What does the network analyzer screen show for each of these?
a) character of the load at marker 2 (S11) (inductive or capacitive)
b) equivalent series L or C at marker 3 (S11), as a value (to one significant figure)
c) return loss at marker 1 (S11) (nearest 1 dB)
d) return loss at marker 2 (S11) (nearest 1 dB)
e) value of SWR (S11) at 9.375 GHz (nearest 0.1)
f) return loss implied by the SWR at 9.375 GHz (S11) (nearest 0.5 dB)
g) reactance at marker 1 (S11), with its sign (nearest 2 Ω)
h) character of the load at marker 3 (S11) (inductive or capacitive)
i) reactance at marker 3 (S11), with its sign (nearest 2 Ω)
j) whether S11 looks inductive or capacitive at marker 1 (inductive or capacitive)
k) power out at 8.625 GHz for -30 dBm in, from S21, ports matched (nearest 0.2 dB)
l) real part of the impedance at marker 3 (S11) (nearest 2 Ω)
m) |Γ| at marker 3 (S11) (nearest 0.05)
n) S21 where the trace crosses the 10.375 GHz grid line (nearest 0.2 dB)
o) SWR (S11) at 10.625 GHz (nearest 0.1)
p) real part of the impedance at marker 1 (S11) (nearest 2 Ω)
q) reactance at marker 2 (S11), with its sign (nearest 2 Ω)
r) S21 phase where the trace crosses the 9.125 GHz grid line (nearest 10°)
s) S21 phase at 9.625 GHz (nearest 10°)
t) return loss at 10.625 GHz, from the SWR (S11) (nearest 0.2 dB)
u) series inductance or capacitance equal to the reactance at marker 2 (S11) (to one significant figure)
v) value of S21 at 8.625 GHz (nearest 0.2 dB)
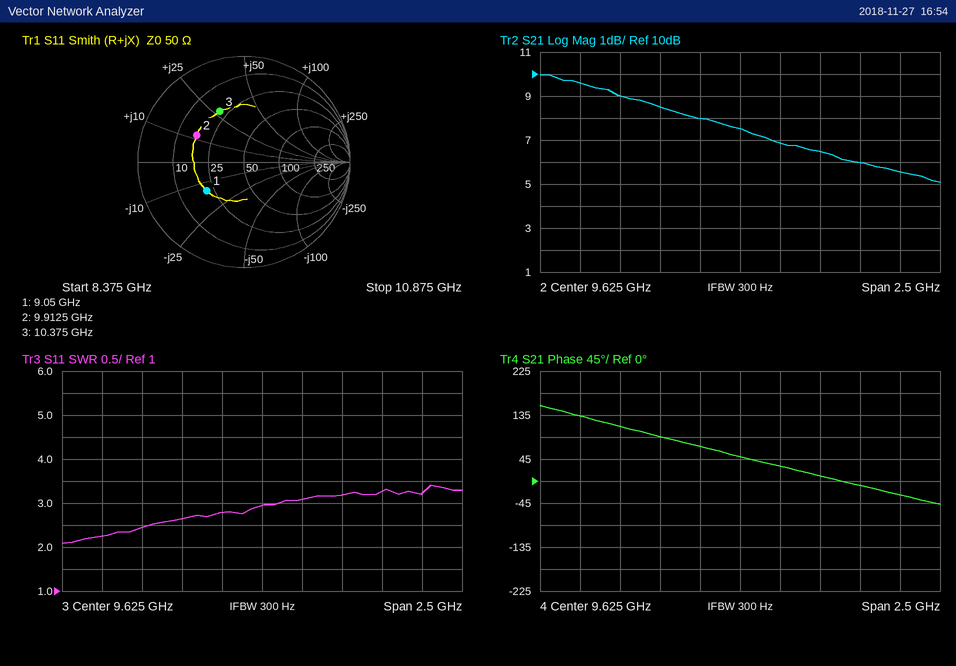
inductive
400 pH
7 dB
6 dB
2.8
6.5 dB
-14 Ω
inductive
+28 Ω
capacitive
-20.4 dBm
20 Ω
0.55
6.0 dB
3.2
22 Ω
+12 Ω
90°
50°
5.6 dB
200 pH
9.6 dB
